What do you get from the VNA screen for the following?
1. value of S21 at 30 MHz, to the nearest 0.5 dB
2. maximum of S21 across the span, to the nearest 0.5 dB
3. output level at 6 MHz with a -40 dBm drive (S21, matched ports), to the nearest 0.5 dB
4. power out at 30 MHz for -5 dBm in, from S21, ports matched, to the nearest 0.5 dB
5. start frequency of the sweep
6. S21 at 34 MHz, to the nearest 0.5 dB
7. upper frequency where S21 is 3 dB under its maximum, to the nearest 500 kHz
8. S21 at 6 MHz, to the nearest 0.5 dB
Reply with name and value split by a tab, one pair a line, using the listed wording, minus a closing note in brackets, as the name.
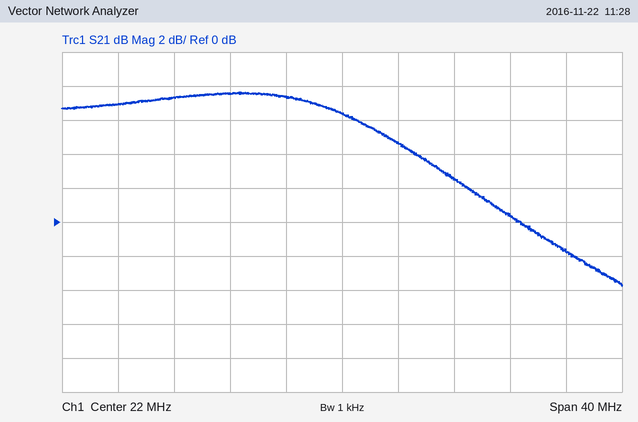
value of S21 at 30 MHz, to the nearest 0.5 dB	2.5 dB
maximum of S21 across the span, to the nearest 0.5 dB	7.5 dB
output level at 6 MHz with a -40 dBm drive (S21, matched ports), to the nearest 0.5 dB	-33.0 dBm
power out at 30 MHz for -5 dBm in, from S21, ports matched, to the nearest 0.5 dB	-2.5 dBm
start frequency of the sweep	2 MHz
S21 at 34 MHz, to the nearest 0.5 dB	0.5 dB
upper frequency where S21 is 3 dB under its maximum, to the nearest 500 kHz	26.0 MHz
S21 at 6 MHz, to the nearest 0.5 dB	7.0 dB
